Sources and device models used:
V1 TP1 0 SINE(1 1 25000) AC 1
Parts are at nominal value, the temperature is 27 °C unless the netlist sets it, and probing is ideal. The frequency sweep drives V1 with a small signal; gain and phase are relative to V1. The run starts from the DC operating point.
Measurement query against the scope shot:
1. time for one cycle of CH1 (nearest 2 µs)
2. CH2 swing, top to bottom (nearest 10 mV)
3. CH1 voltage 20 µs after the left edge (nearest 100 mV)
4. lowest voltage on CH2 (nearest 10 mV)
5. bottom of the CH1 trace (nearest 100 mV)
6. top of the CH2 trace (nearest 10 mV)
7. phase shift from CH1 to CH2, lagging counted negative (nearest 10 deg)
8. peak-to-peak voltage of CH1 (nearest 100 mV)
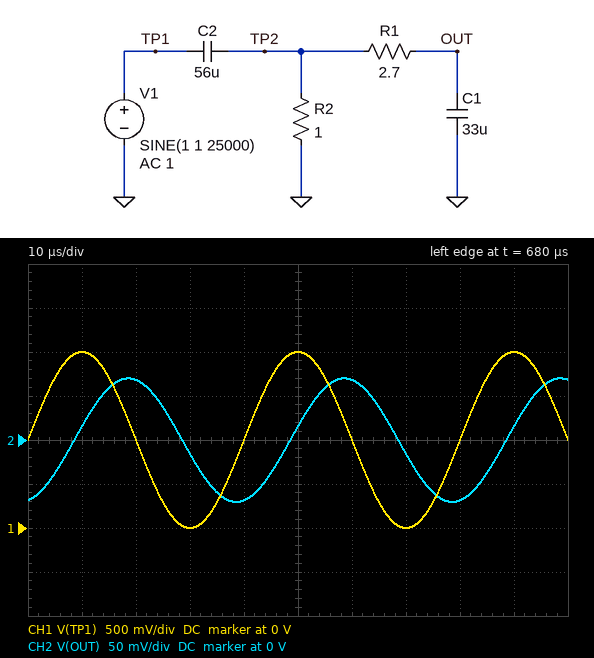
40 µs
140 mV
1.0 V
-70 mV
0 V
70 mV
-80 deg
2.0 V
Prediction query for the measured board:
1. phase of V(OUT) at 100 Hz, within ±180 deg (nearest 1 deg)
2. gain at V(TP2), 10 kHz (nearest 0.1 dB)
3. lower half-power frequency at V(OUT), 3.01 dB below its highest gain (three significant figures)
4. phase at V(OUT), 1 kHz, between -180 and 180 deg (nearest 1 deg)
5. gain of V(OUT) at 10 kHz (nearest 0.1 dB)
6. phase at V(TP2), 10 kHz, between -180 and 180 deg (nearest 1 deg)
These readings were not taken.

84 deg
-0.7 dB
785 Hz
36 deg
-15.8 dB
21 deg
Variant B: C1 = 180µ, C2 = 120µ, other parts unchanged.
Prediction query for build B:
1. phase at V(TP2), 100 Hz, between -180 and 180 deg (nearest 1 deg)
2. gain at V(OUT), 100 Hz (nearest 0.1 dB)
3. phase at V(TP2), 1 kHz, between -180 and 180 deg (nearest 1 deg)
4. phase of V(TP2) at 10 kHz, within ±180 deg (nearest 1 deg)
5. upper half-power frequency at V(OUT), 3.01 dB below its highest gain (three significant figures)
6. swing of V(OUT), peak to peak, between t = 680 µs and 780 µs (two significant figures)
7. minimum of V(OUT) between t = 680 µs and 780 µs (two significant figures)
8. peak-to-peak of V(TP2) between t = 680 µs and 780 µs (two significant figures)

80 deg
-23.2 dB
57 deg
10 deg
2.33 kHz
26 mV
-14 mV
2.0 V
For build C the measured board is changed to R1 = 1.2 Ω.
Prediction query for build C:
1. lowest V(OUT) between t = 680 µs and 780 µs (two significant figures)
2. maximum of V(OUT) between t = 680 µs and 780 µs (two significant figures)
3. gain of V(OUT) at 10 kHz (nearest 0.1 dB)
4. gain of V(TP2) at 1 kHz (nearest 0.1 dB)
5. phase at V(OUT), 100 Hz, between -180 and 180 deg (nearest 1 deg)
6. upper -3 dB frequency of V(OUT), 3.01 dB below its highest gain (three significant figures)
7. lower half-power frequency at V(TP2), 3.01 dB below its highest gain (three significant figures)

-150 mV
150 mV
-10.1 dB
-10.5 dB
85 deg
10.3 kHz
5.82 kHz
